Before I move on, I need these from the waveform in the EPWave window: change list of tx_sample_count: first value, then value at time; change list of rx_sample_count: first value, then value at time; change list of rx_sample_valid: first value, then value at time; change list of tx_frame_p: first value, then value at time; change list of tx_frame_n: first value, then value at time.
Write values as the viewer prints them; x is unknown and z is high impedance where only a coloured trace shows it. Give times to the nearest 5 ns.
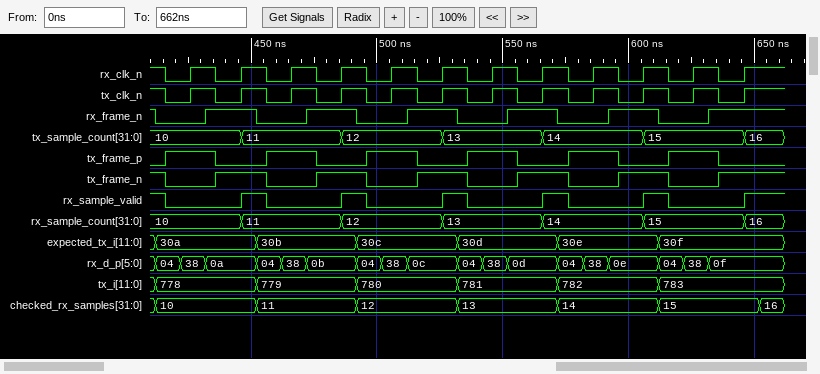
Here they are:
10, 11 at 445 ns, 12 at 485 ns, 13 at 525 ns, 14 at 565 ns, 15 at 605 ns, 16 at 645 ns
10, 11 at 445 ns, 12 at 485 ns, 13 at 525 ns, 14 at 565 ns, 15 at 605 ns, 16 at 645 ns
1, 0 at 415 ns, 1 at 445 ns, 0 at 455 ns, 1 at 485 ns, 0 at 495 ns, 1 at 525 ns, 0 at 535 ns, 1 at 565 ns, 0 at 575 ns, 1 at 605 ns, 0 at 615 ns, 1 at 645 ns
0, 1 at 415 ns, 0 at 435 ns, 1 at 455 ns, 0 at 475 ns, 1 at 495 ns, 0 at 515 ns, 1 at 535 ns, 0 at 555 ns, 1 at 575 ns, 0 at 595 ns, 1 at 615 ns, 0 at 635 ns
1, 0 at 415 ns, 1 at 435 ns, 0 at 455 ns, 1 at 475 ns, 0 at 495 ns, 1 at 515 ns, 0 at 535 ns, 1 at 555 ns, 0 at 575 ns, 1 at 595 ns, 0 at 615 ns, 1 at 635 ns
